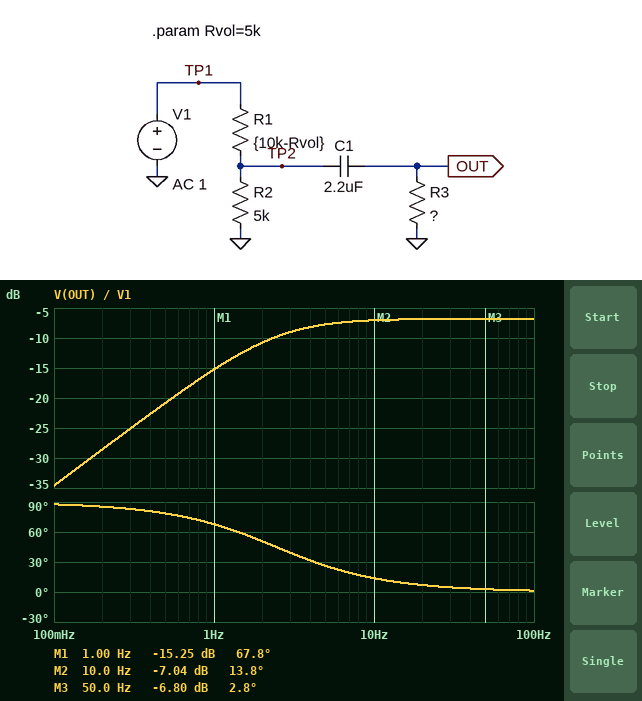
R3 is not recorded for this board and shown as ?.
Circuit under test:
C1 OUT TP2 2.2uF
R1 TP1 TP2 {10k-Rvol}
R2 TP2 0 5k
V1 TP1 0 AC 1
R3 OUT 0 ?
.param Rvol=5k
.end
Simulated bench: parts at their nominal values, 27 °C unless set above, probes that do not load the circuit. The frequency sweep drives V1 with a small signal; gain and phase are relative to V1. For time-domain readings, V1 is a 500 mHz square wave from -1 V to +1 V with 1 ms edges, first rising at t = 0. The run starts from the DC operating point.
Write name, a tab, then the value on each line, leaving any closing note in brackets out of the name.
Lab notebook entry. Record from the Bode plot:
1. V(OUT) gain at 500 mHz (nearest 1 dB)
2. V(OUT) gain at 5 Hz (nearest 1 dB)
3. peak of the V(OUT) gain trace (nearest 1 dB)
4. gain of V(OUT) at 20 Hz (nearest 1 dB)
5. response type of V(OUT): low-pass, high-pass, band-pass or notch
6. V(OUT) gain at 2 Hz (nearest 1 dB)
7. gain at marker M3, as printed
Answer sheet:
V(OUT) gain at 500 mHz	-21 dB
V(OUT) gain at 5 Hz	-8 dB
peak of the V(OUT) gain trace	-7 dB
gain of V(OUT) at 20 Hz	-7 dB
response type of V(OUT): low-pass, high-pass, band-pass or notch	high-pass
V(OUT) gain at 2 Hz	-11 dB
gain at marker M3, as printed	-6.80 dB
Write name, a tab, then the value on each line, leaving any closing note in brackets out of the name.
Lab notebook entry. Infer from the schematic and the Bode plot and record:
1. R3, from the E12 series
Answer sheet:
R3, from the E12 series	27 kΩ
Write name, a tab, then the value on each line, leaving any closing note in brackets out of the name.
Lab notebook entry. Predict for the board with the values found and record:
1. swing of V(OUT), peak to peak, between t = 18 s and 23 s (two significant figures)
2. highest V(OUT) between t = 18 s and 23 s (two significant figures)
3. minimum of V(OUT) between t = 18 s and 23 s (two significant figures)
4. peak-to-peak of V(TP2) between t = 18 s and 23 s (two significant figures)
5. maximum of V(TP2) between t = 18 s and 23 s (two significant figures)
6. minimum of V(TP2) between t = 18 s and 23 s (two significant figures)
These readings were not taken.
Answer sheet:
swing of V(OUT), peak to peak, between t = 18 s and 23 s	1.8 V
highest V(OUT) between t = 18 s and 23 s	910 mV
minimum of V(OUT) between t = 18 s and 23 s	-910 mV
peak-to-peak of V(TP2) between t = 18 s and 23 s	1.0 V
maximum of V(TP2) between t = 18 s and 23 s	500 mV
minimum of V(TP2) between t = 18 s and 23 s	-500 mV
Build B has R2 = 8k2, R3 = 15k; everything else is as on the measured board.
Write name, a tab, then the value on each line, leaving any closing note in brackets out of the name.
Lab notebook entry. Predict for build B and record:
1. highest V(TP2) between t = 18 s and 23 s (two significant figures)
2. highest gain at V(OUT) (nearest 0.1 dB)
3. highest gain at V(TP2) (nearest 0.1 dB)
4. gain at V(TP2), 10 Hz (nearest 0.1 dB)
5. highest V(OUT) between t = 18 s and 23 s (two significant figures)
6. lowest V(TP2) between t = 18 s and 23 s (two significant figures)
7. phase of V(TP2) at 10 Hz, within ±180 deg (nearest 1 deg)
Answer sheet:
highest V(TP2) between t = 18 s and 23 s	620 mV
highest gain at V(OUT)	-5.8 dB
highest gain at V(TP2)	-4.1 dB
gain at V(TP2), 10 Hz	-5.5 dB
highest V(OUT) between t = 18 s and 23 s	1.0 V
lowest V(TP2) between t = 18 s and 23 s	-620 mV
phase of V(TP2) at 10 Hz, within ±180 deg	-4 deg
